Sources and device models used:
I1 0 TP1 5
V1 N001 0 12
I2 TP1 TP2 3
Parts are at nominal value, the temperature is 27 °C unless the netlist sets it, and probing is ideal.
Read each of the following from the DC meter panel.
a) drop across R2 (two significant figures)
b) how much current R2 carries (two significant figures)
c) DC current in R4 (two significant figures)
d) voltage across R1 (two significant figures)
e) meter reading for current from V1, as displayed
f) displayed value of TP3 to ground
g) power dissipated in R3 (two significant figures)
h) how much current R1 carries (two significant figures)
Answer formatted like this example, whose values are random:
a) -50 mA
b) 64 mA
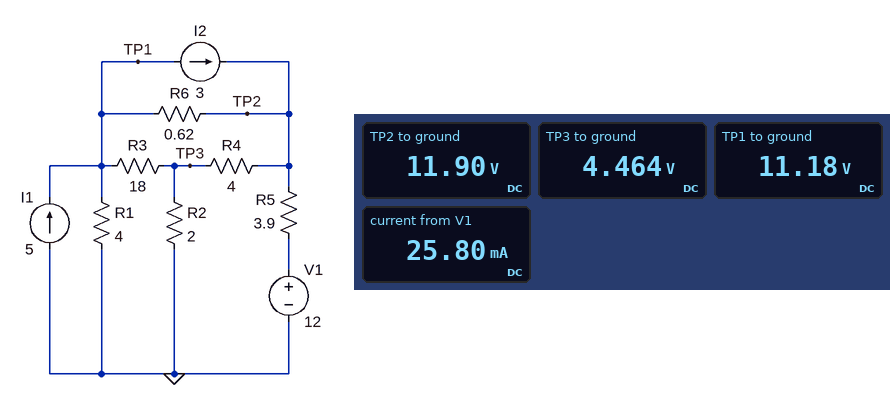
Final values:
a) 4.5 V
b) 2.2 A
c) 1.9 A
d) 11 V
e) 25.80 mA
f) 4.464 V
g) 2.5 W
h) 2.8 A
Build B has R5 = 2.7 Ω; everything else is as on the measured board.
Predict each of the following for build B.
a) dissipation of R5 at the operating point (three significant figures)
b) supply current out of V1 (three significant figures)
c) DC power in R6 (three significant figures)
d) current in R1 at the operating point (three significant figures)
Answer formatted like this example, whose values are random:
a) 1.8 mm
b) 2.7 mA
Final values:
a) 2.72 mW
b) 31.7 mA
c) 849 mW
d) 2.80 A
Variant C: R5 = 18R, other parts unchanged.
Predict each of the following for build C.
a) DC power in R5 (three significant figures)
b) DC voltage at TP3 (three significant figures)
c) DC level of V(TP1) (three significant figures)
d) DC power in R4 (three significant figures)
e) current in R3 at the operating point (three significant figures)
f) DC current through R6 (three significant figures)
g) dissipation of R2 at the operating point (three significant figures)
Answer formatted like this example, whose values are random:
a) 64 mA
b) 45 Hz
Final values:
a) 1.17 mW
b) 4.45 V
c) 11.1 V
d) 13.7 W
e) 372 mA
f) 1.16 A
g) 9.89 W
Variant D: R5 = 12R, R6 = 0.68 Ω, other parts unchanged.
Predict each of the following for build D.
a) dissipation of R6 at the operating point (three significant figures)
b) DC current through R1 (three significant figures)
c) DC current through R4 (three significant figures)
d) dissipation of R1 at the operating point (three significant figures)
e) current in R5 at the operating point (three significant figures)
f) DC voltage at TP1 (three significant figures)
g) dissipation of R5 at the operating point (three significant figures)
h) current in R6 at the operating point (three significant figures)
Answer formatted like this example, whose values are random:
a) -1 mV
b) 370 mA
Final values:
a) 898 mW
b) 2.78 A
c) 1.86 A
d) 30.9 W
e) 8.54 mA
f) 11.1 V
g) 876 µW
h) 1.15 A
